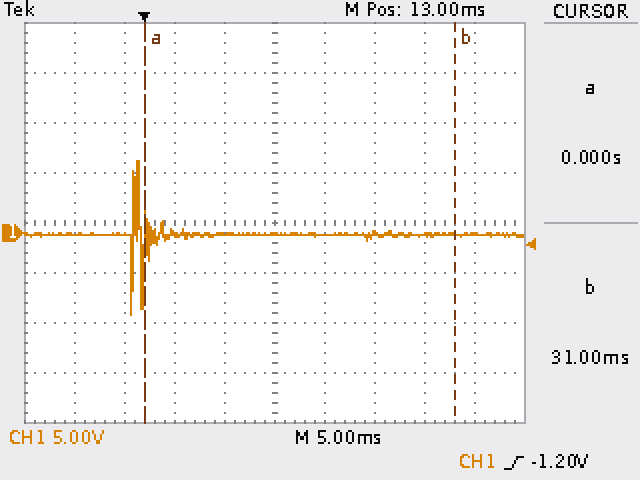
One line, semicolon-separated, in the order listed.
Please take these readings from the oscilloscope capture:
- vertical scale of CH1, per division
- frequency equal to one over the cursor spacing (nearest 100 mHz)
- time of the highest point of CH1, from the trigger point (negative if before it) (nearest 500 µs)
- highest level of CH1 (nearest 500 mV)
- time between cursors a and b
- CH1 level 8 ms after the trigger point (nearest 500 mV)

5 V; 32.3 Hz; -500 µs; 7.0 V; 31.0 ms; 0.0 V
